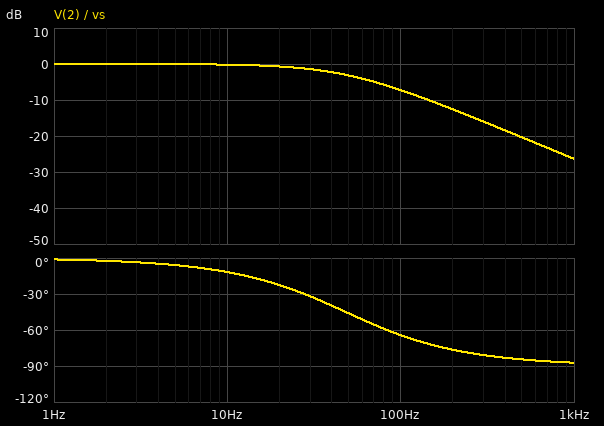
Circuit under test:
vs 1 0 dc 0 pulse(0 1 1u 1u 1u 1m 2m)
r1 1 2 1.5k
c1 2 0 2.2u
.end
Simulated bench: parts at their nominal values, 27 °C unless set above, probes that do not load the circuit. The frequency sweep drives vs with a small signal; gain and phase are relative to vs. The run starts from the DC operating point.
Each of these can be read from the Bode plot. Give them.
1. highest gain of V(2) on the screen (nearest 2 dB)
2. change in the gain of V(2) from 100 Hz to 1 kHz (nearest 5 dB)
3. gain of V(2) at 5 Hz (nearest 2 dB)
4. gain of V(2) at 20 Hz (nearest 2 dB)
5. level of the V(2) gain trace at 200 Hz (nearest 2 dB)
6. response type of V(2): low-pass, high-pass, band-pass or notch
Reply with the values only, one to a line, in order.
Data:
0 dB
-20 dB
0 dB
0 dB
-12 dB
low-pass
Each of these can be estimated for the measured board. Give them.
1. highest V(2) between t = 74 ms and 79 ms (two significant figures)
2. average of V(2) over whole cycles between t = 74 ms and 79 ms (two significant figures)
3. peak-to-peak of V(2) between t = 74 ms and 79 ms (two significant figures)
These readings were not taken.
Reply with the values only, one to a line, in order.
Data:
580 mV
500 mV
150 mV
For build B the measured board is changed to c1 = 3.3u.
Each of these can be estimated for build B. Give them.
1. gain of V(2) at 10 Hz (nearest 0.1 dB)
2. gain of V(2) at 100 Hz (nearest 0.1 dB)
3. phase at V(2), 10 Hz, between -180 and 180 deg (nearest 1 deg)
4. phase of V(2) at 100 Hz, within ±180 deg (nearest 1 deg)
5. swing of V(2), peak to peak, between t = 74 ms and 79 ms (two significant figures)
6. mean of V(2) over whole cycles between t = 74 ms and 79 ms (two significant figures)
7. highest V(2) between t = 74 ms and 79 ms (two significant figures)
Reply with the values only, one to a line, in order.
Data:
-0.4 dB
-10.3 dB
-17 deg
-72 deg
100 mV
500 mV
550 mV
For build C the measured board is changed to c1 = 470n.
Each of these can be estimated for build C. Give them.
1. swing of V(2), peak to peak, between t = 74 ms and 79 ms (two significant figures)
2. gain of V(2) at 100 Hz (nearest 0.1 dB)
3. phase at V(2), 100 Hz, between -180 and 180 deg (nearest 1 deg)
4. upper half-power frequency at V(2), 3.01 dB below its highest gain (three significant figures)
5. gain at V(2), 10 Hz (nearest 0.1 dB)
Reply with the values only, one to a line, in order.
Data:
610 mV
-0.8 dB
-24 deg
226 Hz
0 dB
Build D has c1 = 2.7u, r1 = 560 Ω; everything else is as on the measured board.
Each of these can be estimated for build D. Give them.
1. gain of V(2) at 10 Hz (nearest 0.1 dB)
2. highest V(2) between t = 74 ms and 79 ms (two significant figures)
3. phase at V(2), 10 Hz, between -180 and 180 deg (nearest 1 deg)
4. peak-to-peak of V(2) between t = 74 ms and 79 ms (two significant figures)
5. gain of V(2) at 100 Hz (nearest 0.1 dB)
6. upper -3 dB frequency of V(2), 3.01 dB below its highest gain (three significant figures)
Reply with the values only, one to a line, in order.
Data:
0 dB
660 mV
-5 deg
320 mV
-2.8 dB
105 Hz
